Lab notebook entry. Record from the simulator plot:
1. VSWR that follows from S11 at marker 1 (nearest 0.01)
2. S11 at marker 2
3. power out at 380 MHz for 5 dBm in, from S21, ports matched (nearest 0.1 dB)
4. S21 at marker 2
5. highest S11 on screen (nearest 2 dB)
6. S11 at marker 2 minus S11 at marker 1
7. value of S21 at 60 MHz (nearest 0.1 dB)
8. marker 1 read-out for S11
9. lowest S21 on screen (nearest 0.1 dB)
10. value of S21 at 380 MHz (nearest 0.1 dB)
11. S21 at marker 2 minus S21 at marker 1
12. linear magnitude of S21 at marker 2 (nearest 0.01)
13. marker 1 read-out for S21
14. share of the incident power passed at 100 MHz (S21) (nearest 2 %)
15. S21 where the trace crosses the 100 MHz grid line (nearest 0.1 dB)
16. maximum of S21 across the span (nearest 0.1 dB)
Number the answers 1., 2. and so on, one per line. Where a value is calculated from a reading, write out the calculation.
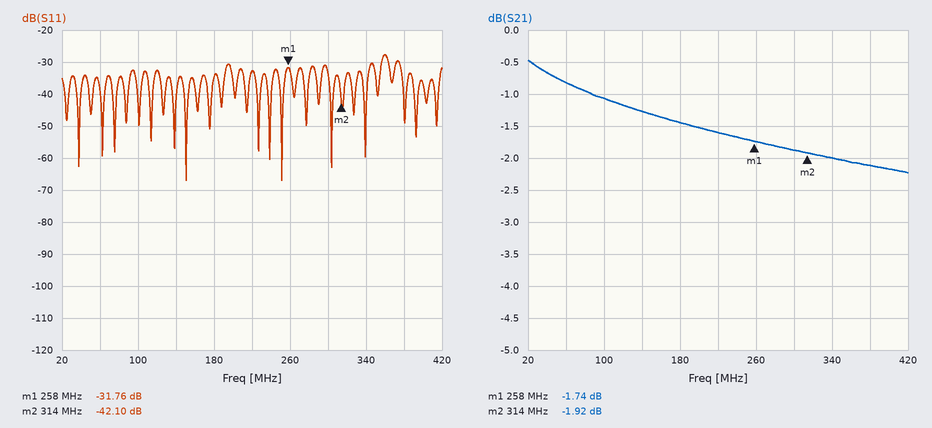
1. (1 + 0.0258)/(1 − 0.0258) ≈ 1.05
2. -42.10 dB
3. 5 dBm + (-2.1 dB) = 2.9 dBm
4. -1.92 dB
5. -28 dB
6. -42.1 − (-31.76) = -10.34 dB
7. -0.8 dB
8. -31.76 dB
9. -2.2 dB
10. -2.1 dB
11. -1.92 − (-1.74) = -0.18 dB
12. 10^(-1.92/20) ≈ 0.80
13. -1.74 dB
14. 10^(-1.1/10) ≈ 78 %
15. -1.1 dB
16. -0.5 dB
